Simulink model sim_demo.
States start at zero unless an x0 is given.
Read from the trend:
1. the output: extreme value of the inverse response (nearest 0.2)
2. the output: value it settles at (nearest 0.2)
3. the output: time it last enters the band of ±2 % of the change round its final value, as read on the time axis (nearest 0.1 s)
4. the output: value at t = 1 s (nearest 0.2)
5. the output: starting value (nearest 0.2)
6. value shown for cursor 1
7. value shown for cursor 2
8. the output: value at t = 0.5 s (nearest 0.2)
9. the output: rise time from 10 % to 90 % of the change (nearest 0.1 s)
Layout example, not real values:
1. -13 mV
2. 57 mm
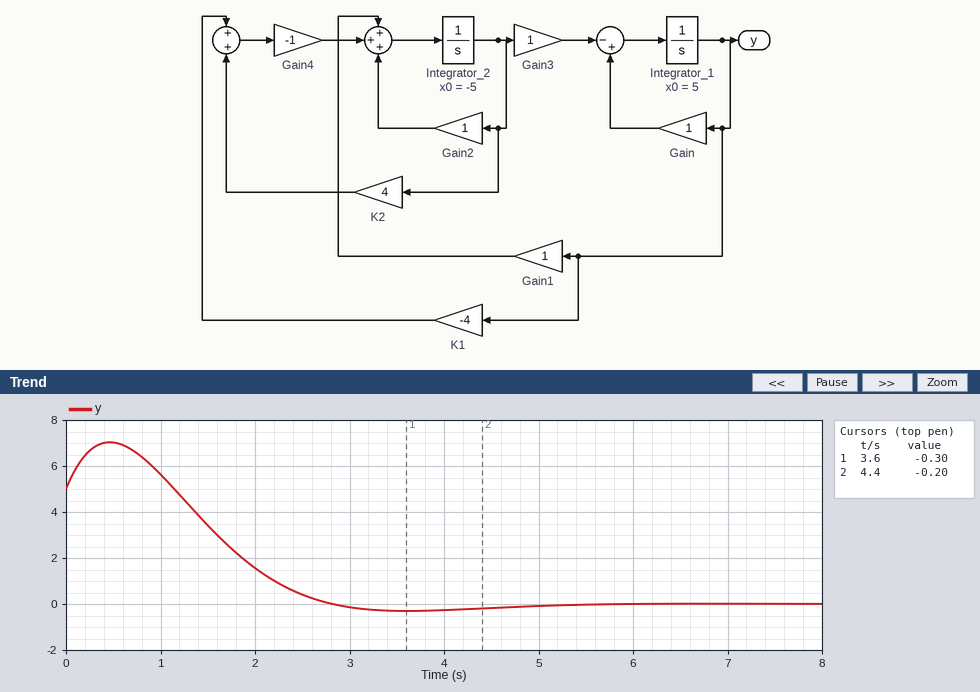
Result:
1. 7.0
2. 0.0
3. 4.9 s
4. 5.6
5. 5.0
6. -0.30
7. -0.20
8. 7.0
9. 1.2 s
